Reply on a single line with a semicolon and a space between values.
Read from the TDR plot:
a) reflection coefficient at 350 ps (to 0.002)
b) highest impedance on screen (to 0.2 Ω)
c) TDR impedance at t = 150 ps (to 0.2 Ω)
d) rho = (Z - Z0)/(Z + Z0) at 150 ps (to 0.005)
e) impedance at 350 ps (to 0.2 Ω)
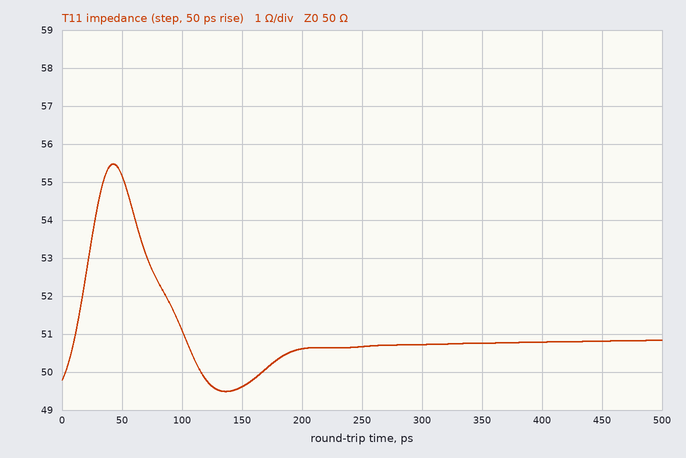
+0.008; 55.4 Ω; 49.6 Ω; -0.005; 50.8 Ω
